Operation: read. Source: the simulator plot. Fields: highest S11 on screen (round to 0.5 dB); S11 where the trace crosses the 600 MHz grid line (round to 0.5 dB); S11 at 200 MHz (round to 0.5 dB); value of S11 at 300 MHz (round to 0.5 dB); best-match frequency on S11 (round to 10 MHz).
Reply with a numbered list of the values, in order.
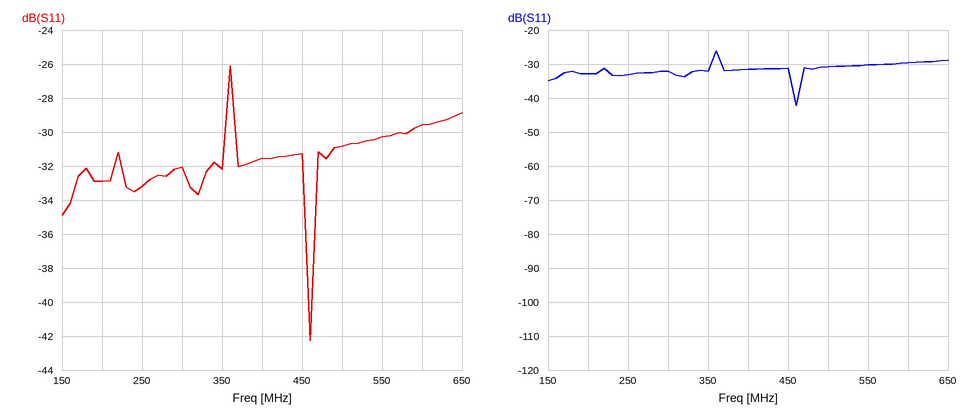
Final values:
1. -26.0 dB
2. -29.5 dB
3. -33.0 dB
4. -32.0 dB
5. 460 MHz
